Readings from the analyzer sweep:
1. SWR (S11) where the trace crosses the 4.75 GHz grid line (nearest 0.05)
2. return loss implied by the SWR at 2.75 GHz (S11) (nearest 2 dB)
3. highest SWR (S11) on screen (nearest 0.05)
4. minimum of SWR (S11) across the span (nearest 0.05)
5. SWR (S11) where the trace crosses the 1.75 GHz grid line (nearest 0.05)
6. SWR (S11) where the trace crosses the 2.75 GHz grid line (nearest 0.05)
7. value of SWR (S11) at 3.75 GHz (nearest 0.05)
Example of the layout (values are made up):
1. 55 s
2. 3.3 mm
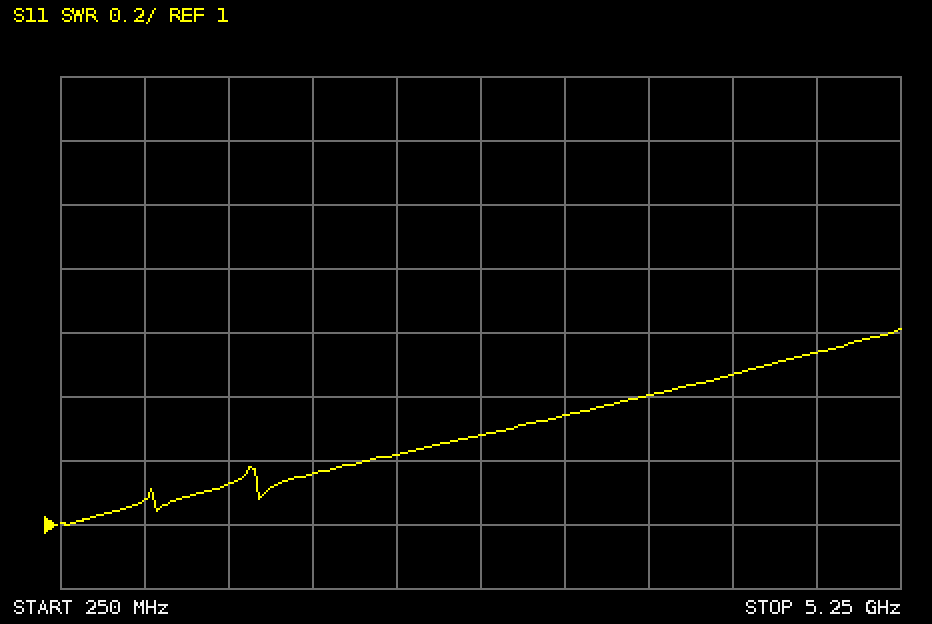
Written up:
1. 1.55
2. 18 dB
3. 1.60
4. 1.00
5. 1.15
6. 1.30
7. 1.40
